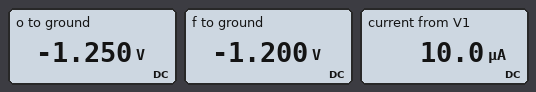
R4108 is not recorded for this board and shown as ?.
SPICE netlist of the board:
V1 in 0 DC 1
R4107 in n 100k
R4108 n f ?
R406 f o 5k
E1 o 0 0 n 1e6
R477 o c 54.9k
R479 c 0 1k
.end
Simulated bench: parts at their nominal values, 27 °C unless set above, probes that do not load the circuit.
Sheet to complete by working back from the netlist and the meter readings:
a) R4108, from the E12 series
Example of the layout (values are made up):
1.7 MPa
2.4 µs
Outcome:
120 kΩ
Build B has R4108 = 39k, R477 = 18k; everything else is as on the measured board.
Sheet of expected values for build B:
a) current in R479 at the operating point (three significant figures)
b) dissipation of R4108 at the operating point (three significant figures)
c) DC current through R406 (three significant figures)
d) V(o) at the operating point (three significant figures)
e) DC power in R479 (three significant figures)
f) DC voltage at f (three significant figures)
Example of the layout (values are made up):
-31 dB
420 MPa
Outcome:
23.2 µA
3.90 µW
10.0 µA
-440 mV
536 nW
-390 mV
